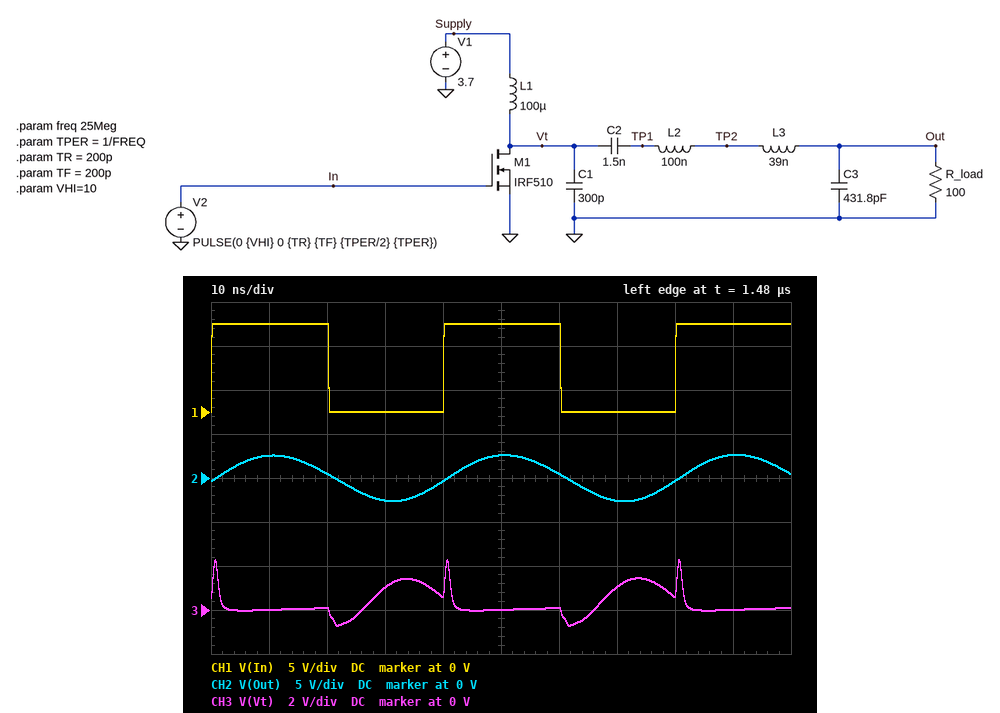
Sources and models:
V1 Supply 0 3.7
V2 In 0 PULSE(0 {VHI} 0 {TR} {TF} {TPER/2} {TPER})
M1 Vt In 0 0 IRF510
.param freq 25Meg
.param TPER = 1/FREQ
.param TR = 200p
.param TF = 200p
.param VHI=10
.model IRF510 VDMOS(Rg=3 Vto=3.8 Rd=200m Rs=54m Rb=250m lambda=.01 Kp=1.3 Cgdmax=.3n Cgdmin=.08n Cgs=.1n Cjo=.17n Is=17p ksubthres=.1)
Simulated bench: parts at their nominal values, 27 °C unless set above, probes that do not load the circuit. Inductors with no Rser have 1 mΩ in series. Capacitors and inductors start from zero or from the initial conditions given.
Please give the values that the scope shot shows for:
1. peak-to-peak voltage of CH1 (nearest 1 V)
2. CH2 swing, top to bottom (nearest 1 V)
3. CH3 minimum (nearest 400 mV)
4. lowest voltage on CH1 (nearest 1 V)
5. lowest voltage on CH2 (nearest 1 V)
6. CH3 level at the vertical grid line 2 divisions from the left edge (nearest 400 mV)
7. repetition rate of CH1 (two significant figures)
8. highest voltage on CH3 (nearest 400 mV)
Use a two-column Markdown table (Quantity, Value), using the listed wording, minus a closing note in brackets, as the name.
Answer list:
| Quantity | Value |
|---|---|
| peak-to-peak voltage of CH1 | 10 V |
| CH2 swing, top to bottom | 5 V |
| CH3 minimum | -800 mV |
| lowest voltage on CH1 | 0 V |
| lowest voltage on CH2 | -3 V |
| CH3 level at the vertical grid line 2 divisions from the left edge | 0 V |
| repetition rate of CH1 | 25 MHz |
| highest voltage on CH3 | 2.4 V |
